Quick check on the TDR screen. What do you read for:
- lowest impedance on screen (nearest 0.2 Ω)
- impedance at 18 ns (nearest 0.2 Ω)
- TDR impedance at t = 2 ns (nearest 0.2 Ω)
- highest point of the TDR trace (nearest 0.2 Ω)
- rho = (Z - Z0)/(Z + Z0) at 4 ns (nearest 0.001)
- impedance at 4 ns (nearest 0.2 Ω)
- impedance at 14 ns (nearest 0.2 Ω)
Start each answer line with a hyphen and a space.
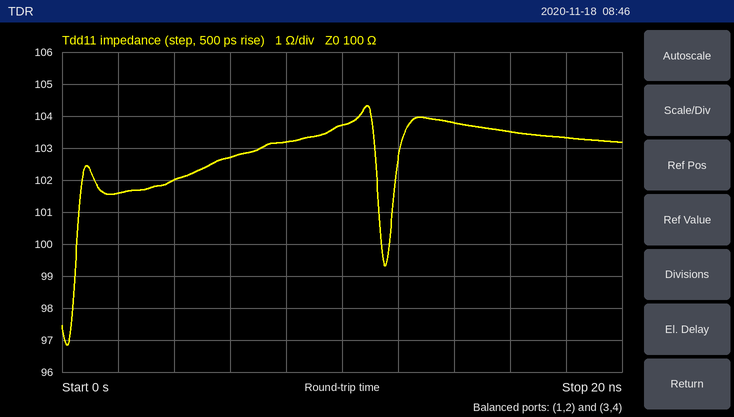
- 96.8 Ω
- 103.4 Ω
- 101.6 Ω
- 104.4 Ω
- +0.010
- 102.0 Ω
- 103.8 Ω
